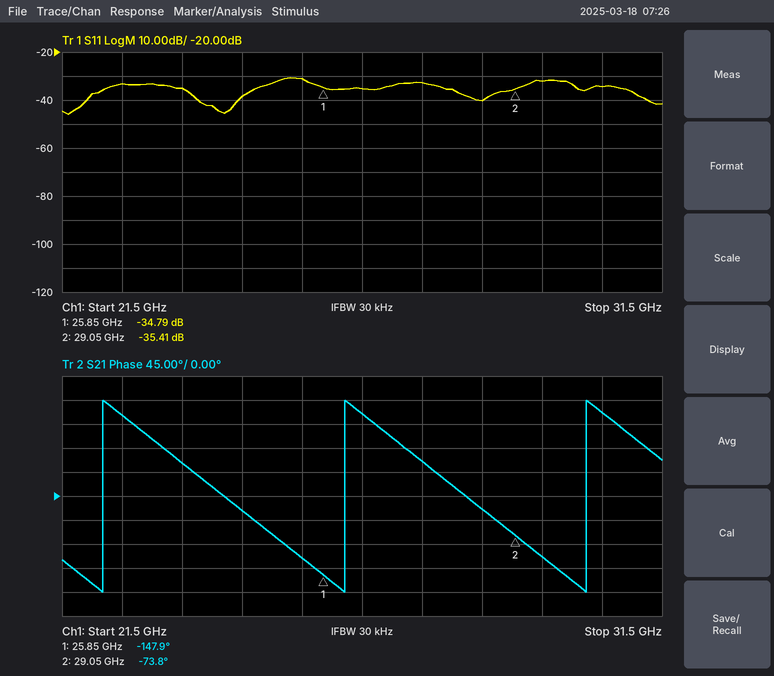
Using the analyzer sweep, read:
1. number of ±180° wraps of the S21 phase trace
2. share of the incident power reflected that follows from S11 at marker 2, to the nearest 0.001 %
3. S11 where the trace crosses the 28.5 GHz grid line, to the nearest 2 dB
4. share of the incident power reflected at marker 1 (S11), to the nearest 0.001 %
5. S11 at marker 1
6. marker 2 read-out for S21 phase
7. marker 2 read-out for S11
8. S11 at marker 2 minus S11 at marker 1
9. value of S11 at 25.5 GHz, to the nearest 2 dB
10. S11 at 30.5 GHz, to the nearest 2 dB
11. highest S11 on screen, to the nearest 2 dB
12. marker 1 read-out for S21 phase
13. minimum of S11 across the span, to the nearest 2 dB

3
0.029 %
-40 dB
0.033 %
-34.79 dB
-73.8°
-35.41 dB
-0.62 dB
-32 dB
-34 dB
-30 dB
-147.9°
-46 dB
